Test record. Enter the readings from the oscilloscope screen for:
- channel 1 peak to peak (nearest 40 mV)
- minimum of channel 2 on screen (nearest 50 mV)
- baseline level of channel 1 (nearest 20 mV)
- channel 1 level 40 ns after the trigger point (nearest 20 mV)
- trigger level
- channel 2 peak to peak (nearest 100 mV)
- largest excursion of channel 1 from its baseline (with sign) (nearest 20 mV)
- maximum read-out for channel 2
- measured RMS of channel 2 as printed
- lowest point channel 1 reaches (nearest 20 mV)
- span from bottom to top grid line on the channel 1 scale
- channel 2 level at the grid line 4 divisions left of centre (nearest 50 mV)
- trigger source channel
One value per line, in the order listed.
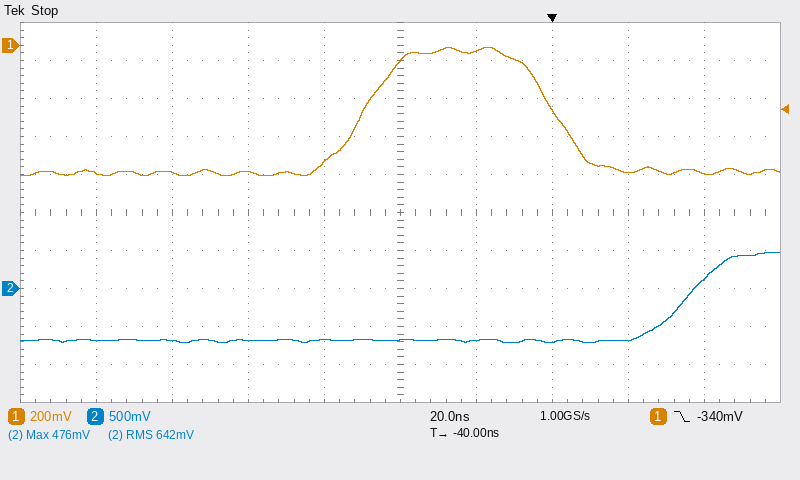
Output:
680 mV
-700 mV
-660 mV
-680 mV
-340 mV
1.20 V
+660 mV
476 mV
642 mV
-680 mV
2 V
-700 mV
channel 1
